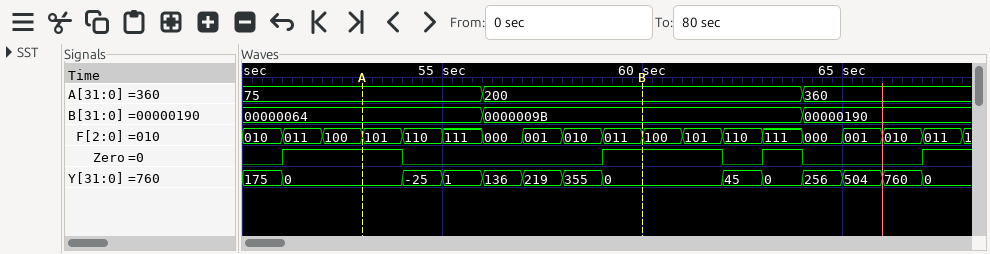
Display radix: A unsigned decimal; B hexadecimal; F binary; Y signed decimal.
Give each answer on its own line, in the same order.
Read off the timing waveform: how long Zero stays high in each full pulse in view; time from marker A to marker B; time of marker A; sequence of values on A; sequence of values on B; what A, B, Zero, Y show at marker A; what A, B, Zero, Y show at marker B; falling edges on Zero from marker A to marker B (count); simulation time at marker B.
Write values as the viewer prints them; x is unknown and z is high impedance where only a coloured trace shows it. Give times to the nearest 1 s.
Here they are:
3 s, 3 s, 1 s
7 s
53 s
75, 200, 360
00000064, 0000009B, 00000190
A=75, B=00000064, Zero=1, Y=0
A=200, B=0000009B, Zero=1, Y=0
1
60 s
